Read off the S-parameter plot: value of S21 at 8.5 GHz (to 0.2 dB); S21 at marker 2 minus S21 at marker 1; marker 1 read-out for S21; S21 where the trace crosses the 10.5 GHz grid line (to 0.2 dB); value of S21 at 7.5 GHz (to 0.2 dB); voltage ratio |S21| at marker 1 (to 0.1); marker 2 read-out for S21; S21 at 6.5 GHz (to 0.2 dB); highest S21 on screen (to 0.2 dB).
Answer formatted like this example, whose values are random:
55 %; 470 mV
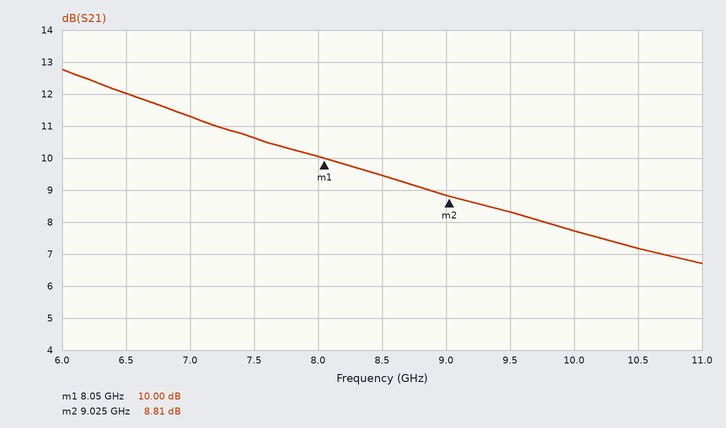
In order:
9.4 dB; -1.19 dB; 10.00 dB; 7.2 dB; 10.6 dB; 3.2; 8.81 dB; 12.0 dB; 12.8 dB
